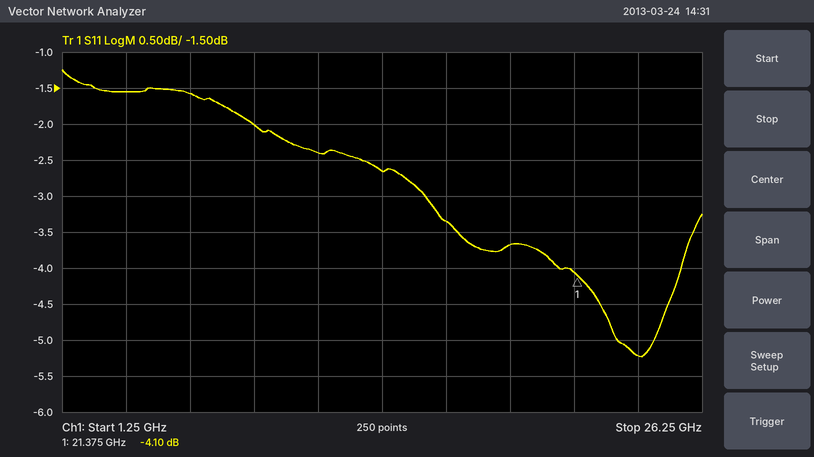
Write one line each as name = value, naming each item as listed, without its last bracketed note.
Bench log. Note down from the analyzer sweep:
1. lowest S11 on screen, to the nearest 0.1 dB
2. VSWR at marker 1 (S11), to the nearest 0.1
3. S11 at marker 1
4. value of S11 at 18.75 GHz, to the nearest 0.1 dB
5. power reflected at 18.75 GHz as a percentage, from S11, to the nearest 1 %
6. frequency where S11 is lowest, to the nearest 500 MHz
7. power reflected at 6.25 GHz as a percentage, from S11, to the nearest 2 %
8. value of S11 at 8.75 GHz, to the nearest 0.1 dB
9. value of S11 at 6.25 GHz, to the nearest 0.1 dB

lowest S11 on screen, to the nearest 0.1 dB = -5.2 dB
VSWR at marker 1 (S11), to the nearest 0.1 = 4.3
S11 at marker 1 = -4.10 dB
value of S11 at 18.75 GHz, to the nearest 0.1 dB = -3.7 dB
power reflected at 18.75 GHz as a percentage, from S11, to the nearest 1 % = 43 %
frequency where S11 is lowest, to the nearest 500 MHz = 24.0 GHz
power reflected at 6.25 GHz as a percentage, from S11, to the nearest 2 % = 70 %
value of S11 at 8.75 GHz, to the nearest 0.1 dB = -2.0 dB
value of S11 at 6.25 GHz, to the nearest 0.1 dB = -1.6 dB
